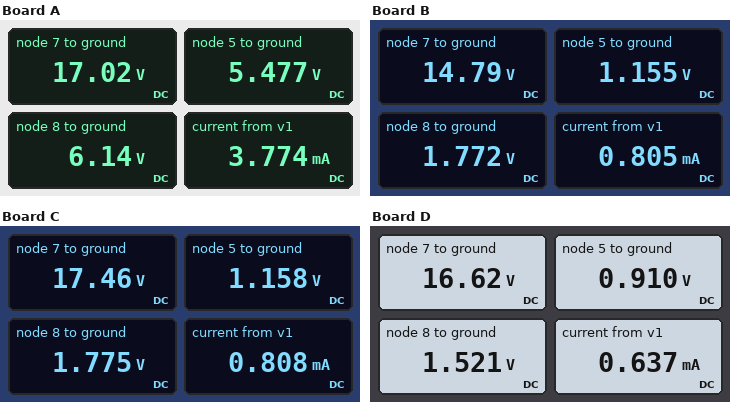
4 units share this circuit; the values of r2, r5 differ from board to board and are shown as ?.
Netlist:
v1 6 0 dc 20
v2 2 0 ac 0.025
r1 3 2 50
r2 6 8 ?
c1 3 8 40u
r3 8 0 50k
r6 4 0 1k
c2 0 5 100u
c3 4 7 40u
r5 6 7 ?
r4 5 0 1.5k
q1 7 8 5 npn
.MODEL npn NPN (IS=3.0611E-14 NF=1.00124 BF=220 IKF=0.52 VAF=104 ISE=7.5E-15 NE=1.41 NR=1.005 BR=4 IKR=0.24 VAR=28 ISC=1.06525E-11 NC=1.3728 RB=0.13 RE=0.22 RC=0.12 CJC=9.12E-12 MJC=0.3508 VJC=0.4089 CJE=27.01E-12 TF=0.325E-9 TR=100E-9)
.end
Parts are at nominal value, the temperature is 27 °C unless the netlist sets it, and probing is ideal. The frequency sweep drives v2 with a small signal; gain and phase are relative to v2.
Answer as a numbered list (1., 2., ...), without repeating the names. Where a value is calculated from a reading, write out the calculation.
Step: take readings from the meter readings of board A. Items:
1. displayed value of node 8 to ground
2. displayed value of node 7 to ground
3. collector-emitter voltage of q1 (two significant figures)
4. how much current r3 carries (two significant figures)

1. 6.14 V
2. 17.02 V
3. 17.02 V - 5.477 V = 12 V
4. (6.14 V) / 50 kΩ = 120 µA
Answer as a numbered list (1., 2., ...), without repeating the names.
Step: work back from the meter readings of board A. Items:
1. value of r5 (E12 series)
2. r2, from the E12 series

1. 820 Ω
2. 100 kΩ
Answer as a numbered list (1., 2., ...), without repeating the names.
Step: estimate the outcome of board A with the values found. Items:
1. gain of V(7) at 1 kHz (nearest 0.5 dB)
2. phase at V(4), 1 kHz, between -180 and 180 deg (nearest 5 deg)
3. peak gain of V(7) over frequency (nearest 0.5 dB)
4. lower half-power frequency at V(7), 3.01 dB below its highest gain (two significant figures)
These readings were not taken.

1. 35.0 dB
2. -170 deg
3. 35.5 dB
4. 210 Hz
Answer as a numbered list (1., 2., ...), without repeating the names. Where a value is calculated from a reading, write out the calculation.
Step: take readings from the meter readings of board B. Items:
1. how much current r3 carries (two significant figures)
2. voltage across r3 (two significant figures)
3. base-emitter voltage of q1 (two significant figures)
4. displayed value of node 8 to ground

1. (1.772 V) / 50 kΩ = 35 µA
2. 1.772 V = 1.8 V
3. 1.772 V - 1.155 V = 620 mV
4. 1.772 V
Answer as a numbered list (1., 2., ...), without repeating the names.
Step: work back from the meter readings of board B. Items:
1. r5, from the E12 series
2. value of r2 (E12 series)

1. 6.8 kΩ
2. 470 kΩ
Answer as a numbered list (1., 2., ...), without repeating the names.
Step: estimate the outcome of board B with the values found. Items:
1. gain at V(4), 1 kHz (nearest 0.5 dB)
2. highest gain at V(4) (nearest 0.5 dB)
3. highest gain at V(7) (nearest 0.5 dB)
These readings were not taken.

1. 28.0 dB
2. 28.0 dB
3. 28.0 dB
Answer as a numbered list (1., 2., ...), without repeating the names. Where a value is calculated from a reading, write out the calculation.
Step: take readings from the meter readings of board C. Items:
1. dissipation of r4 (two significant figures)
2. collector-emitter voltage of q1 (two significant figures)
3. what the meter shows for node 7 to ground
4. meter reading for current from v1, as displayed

1. (1.158 V)^2 / 1.5 kΩ = 890 µW
2. 17.46 V - 1.158 V = 16 V
3. 17.46 V
4. 0.808 mA
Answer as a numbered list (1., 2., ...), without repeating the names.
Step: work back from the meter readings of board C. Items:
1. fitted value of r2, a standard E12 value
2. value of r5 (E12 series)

1. 470 kΩ
2. 3.3 kΩ
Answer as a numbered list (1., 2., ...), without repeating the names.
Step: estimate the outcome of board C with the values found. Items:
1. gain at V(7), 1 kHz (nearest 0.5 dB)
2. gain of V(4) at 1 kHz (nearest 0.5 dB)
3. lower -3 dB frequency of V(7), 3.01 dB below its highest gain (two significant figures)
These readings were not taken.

1. 27.0 dB
2. 27.0 dB
3. 48 Hz
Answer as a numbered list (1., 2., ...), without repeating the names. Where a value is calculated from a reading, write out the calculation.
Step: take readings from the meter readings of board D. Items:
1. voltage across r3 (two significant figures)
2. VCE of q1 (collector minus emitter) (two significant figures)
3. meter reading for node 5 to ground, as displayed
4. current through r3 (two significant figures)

1. 1.521 V = 1.5 V
2. 16.62 V - 910 mV = 16 V
3. 0.910 V
4. (1.521 V) / 50 kΩ = 30 µA
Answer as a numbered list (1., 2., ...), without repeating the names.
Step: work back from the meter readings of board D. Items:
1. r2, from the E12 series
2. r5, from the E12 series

1. 560 kΩ
2. 5.6 kΩ
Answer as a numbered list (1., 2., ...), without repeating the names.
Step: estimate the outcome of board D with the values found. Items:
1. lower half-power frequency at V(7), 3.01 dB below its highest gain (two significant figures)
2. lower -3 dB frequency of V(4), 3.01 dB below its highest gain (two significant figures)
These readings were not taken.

1. 38 Hz
2. 38 Hz
